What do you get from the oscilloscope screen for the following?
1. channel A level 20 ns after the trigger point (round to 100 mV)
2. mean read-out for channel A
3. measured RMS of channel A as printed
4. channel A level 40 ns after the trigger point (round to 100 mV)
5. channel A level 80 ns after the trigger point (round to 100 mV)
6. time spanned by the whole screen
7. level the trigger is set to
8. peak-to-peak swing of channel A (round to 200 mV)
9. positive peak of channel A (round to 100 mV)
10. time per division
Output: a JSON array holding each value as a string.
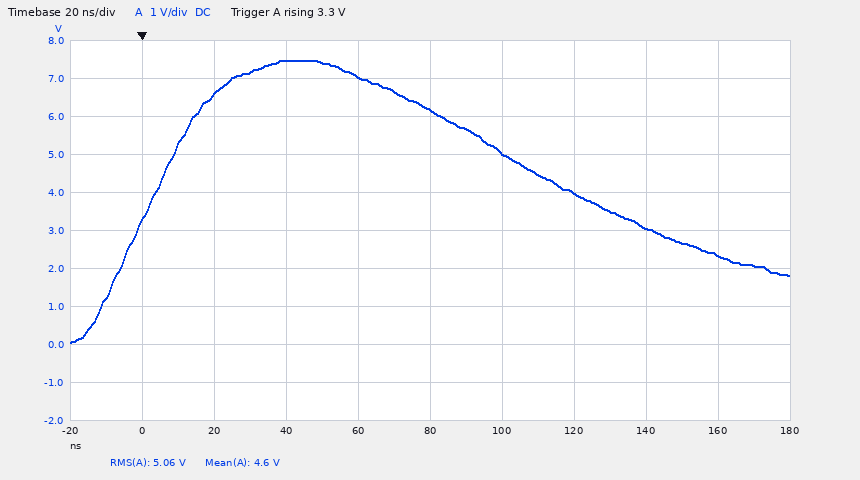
["6.6 V", "4.6 V", "5.06 V", "7.5 V", "6.2 V", "200 ns", "3.3 V", "7.4 V", "7.5 V", "20 ns"]
